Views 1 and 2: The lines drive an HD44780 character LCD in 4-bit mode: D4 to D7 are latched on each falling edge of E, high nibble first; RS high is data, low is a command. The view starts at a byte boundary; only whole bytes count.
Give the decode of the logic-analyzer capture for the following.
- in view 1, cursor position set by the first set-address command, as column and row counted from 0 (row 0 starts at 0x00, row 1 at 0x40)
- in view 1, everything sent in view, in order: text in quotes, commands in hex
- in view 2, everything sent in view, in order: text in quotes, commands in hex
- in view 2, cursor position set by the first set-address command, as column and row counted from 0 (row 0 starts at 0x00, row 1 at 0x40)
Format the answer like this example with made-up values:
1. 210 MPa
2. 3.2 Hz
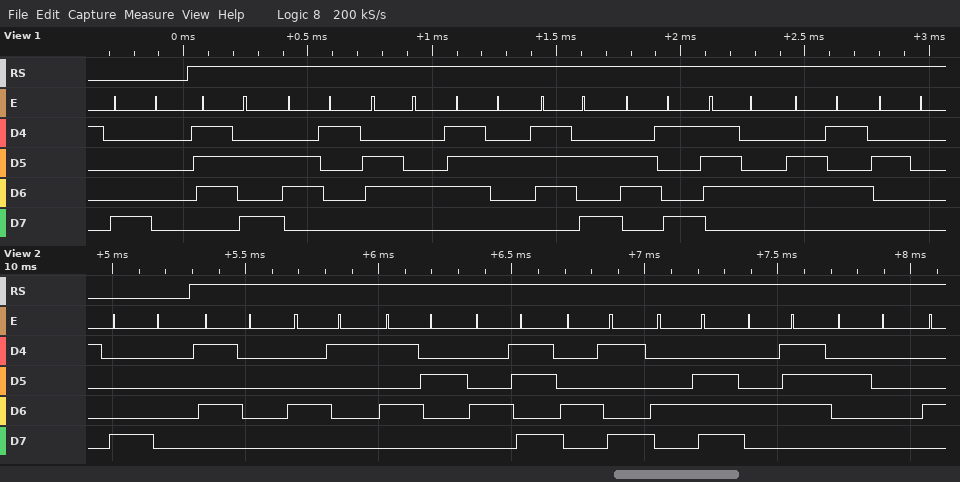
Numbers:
1. column 0, row 0
2. 0x80 "zadrzite "
3. 0x80 "PARKING "
4. column 0, row 0
